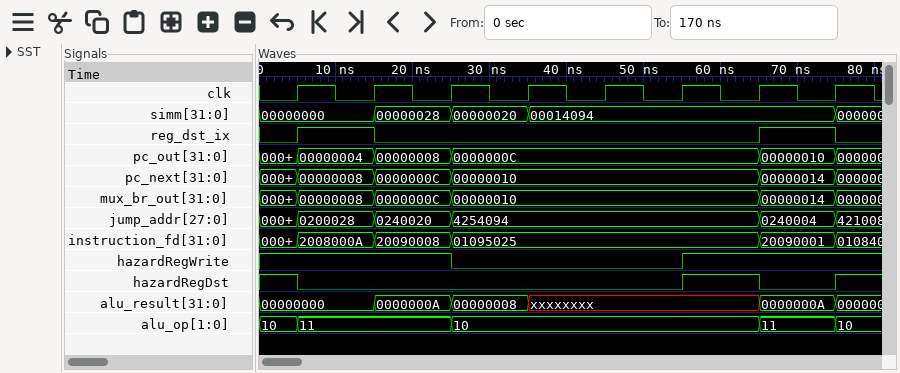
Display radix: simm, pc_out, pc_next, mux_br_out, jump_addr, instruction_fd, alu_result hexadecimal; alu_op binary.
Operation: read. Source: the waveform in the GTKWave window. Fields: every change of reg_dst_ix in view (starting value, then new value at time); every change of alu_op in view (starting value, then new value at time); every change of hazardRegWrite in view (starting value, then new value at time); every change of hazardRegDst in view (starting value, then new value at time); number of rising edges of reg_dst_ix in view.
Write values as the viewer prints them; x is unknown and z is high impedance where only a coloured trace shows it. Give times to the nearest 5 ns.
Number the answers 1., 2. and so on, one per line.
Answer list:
1. 0, 1 at 5 ns, 0 at 15 ns, 1 at 65 ns, 0 at 75 ns
2. 10, 11 at 5 ns, 10 at 25 ns, 11 at 65 ns, 10 at 75 ns
3. 1, 0 at 25 ns, 1 at 55 ns
4. 1, 0 at 5 ns, 1 at 55 ns, 0 at 65 ns, 1 at 75 ns
5. 2
